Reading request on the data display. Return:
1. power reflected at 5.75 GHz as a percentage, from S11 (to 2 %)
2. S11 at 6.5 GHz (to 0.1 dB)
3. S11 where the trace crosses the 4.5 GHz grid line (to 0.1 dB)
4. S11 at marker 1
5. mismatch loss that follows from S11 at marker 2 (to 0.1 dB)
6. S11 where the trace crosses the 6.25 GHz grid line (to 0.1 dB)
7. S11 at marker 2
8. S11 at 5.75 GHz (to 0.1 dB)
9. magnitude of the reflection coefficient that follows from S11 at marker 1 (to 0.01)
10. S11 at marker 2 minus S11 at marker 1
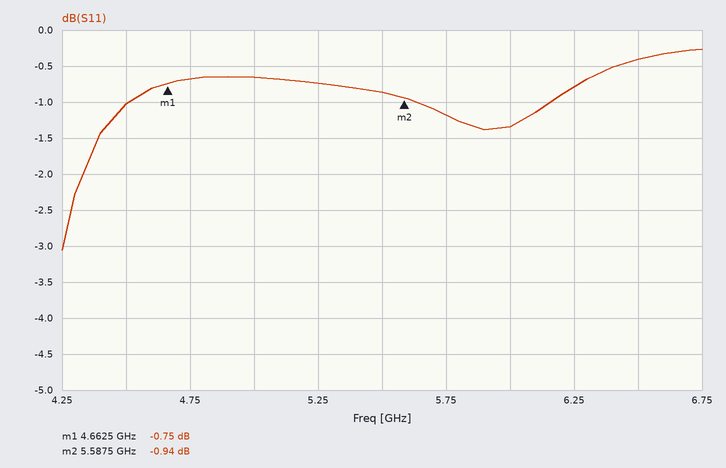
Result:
76 %
-0.4 dB
-1.0 dB
-0.75 dB
7.1 dB
-0.8 dB
-0.94 dB
-1.2 dB
0.92
-0.19 dB
